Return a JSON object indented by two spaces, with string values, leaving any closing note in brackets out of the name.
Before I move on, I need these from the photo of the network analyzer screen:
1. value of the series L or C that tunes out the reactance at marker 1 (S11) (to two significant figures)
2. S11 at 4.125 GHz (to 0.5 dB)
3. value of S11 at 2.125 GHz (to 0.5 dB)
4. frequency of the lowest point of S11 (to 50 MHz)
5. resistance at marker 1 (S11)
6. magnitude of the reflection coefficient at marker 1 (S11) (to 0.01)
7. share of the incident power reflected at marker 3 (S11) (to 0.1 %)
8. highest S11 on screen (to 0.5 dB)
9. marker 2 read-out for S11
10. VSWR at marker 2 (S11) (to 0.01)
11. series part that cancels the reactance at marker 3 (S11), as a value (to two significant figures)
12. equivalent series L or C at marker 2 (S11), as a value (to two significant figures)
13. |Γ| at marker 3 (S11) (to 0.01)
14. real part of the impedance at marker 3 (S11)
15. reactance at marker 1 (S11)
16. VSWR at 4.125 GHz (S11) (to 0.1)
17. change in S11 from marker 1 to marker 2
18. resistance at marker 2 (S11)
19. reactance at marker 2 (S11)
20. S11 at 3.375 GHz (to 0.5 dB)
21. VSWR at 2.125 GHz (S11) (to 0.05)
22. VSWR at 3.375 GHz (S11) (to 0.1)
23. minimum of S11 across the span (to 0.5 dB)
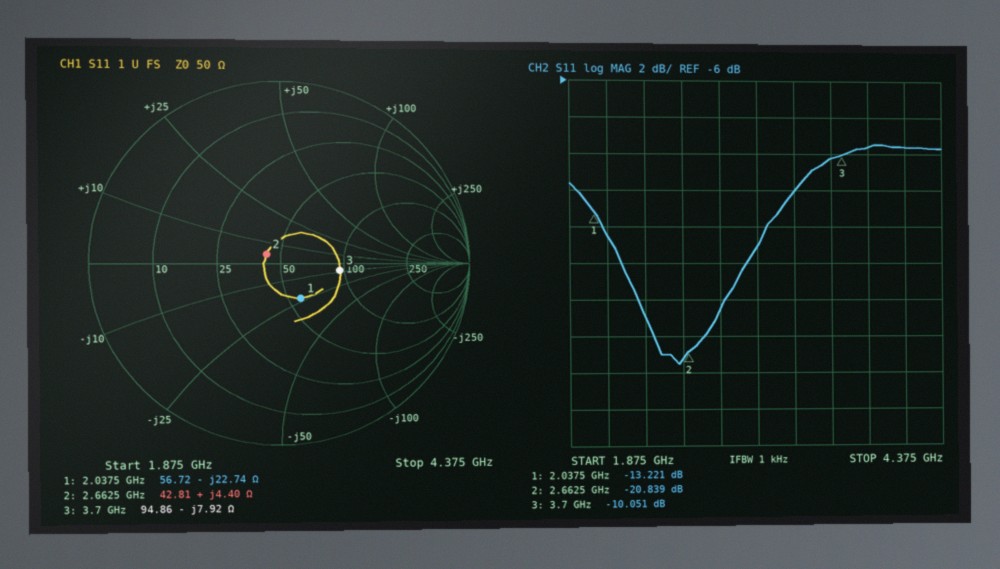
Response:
{
  "value of the series L or C that tunes out the reactance at marker 1 (S11)": "1.8 nH",
  "S11 at 4.125 GHz": "-9.5 dB",
  "value of S11 at 2.125 GHz": "-14.5 dB",
  "frequency of the lowest point of S11": "2.60 GHz",
  "resistance at marker 1": "56.72 Ω",
  "magnitude of the reflection coefficient at marker 1 (S11)": "0.22",
  "share of the incident power reflected at marker 3 (S11)": "9.9 %",
  "highest S11 on screen": "-9.5 dB",
  "marker 2 read-out for S11": "-20.839 dB",
  "VSWR at marker 2 (S11)": "1.20",
  "series part that cancels the reactance at marker 3 (S11), as a value": "340 pH",
  "equivalent series L or C at marker 2 (S11), as a value": "260 pH",
  "|Γ| at marker 3 (S11)": "0.31",
  "real part of the impedance at marker 3": "94.86 Ω",
  "reactance at marker 1": "-22.74 Ω",
  "VSWR at 4.125 GHz (S11)": "2.0",
  "change in S11 from marker 1 to marker 2": "-7.618 dB",
  "resistance at marker 2": "42.81 Ω",
  "reactance at marker 2": "+4.40 Ω",
  "S11 at 3.375 GHz": "-12.0 dB",
  "VSWR at 2.125 GHz (S11)": "1.45",
  "VSWR at 3.375 GHz (S11)": "1.7",
  "minimum of S11 across the span": "-21.5 dB"
}
